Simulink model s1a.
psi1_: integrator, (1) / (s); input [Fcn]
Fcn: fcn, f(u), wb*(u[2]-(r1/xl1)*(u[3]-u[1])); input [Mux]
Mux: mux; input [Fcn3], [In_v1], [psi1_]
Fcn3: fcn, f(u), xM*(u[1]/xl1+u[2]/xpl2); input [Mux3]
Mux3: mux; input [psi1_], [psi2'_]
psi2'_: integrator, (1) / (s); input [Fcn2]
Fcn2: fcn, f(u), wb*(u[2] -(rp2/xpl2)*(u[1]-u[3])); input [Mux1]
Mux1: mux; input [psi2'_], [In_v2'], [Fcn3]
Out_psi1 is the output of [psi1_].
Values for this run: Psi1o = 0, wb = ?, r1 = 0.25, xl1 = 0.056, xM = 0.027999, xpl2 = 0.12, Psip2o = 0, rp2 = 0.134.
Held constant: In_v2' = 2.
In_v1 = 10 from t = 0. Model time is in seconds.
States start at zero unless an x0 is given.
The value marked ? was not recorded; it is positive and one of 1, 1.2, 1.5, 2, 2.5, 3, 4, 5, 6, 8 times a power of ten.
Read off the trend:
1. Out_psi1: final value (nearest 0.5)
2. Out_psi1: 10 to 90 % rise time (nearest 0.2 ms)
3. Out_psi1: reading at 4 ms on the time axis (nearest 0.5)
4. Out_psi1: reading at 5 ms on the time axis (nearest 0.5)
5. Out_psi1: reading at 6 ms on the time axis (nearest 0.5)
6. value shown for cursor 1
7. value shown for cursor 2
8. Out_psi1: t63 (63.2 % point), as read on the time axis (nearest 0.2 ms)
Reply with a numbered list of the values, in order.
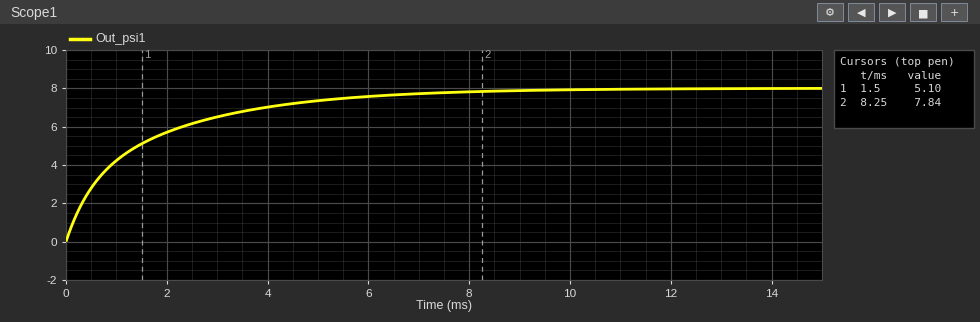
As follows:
1. 8.0
2. 4.4 ms
3. 7.0
4. 7.5
5. 7.5
6. 5.10
7. 7.84
8. 1.4 ms
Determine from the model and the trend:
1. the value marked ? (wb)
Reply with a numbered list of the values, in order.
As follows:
1. 800
